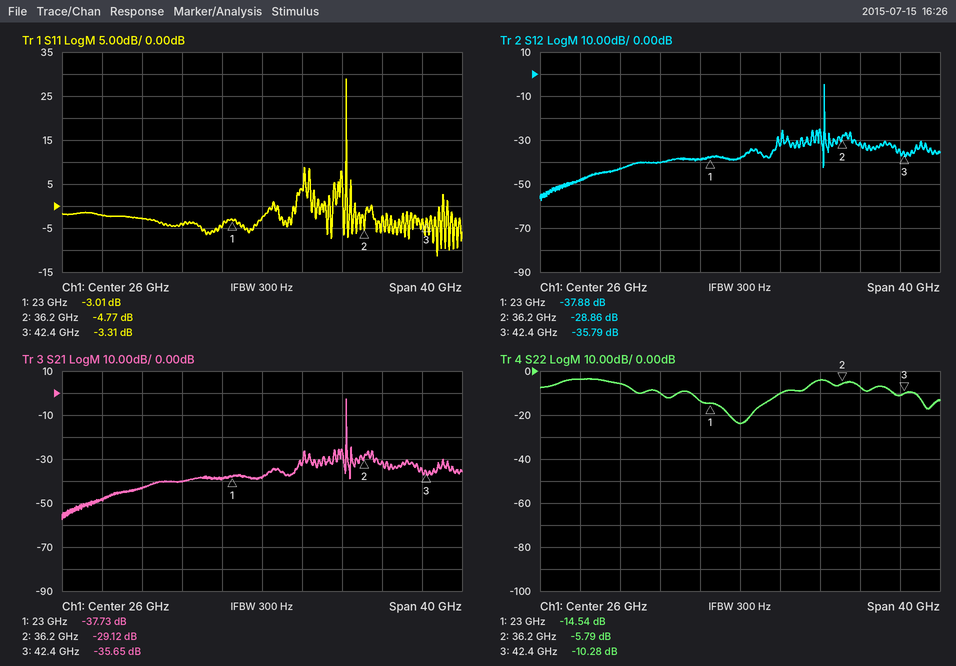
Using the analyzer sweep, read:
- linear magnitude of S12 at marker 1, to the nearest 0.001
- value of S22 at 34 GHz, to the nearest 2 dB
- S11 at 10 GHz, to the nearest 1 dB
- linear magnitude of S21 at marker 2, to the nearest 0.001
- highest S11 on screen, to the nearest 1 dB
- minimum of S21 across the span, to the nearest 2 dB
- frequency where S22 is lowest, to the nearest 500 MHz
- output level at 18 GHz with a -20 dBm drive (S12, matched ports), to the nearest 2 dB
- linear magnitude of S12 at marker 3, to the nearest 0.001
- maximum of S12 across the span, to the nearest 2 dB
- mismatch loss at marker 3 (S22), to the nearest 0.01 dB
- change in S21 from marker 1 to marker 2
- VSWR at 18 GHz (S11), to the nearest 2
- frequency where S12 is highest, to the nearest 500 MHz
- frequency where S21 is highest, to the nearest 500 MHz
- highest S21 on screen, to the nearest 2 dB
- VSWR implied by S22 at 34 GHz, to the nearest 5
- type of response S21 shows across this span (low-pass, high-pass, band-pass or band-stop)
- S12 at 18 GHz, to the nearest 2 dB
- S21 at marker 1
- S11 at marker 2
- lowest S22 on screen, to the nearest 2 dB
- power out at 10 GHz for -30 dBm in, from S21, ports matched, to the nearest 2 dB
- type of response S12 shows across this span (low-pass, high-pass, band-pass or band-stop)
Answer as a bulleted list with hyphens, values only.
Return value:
- 0.013
- -4 dB
- -2 dB
- 0.035
- 29 dB
- -58 dB
- 26.0 GHz
- -60 dBm
- 0.016
- -4 dB
- 0.43 dB
- 8.61 dB
- 4
- 34.5 GHz
- 34.5 GHz
- -2 dB
- 5
- band-pass
- -40 dB
- -37.73 dB
- -4.77 dB
- -24 dB
- -78 dBm
- band-pass
